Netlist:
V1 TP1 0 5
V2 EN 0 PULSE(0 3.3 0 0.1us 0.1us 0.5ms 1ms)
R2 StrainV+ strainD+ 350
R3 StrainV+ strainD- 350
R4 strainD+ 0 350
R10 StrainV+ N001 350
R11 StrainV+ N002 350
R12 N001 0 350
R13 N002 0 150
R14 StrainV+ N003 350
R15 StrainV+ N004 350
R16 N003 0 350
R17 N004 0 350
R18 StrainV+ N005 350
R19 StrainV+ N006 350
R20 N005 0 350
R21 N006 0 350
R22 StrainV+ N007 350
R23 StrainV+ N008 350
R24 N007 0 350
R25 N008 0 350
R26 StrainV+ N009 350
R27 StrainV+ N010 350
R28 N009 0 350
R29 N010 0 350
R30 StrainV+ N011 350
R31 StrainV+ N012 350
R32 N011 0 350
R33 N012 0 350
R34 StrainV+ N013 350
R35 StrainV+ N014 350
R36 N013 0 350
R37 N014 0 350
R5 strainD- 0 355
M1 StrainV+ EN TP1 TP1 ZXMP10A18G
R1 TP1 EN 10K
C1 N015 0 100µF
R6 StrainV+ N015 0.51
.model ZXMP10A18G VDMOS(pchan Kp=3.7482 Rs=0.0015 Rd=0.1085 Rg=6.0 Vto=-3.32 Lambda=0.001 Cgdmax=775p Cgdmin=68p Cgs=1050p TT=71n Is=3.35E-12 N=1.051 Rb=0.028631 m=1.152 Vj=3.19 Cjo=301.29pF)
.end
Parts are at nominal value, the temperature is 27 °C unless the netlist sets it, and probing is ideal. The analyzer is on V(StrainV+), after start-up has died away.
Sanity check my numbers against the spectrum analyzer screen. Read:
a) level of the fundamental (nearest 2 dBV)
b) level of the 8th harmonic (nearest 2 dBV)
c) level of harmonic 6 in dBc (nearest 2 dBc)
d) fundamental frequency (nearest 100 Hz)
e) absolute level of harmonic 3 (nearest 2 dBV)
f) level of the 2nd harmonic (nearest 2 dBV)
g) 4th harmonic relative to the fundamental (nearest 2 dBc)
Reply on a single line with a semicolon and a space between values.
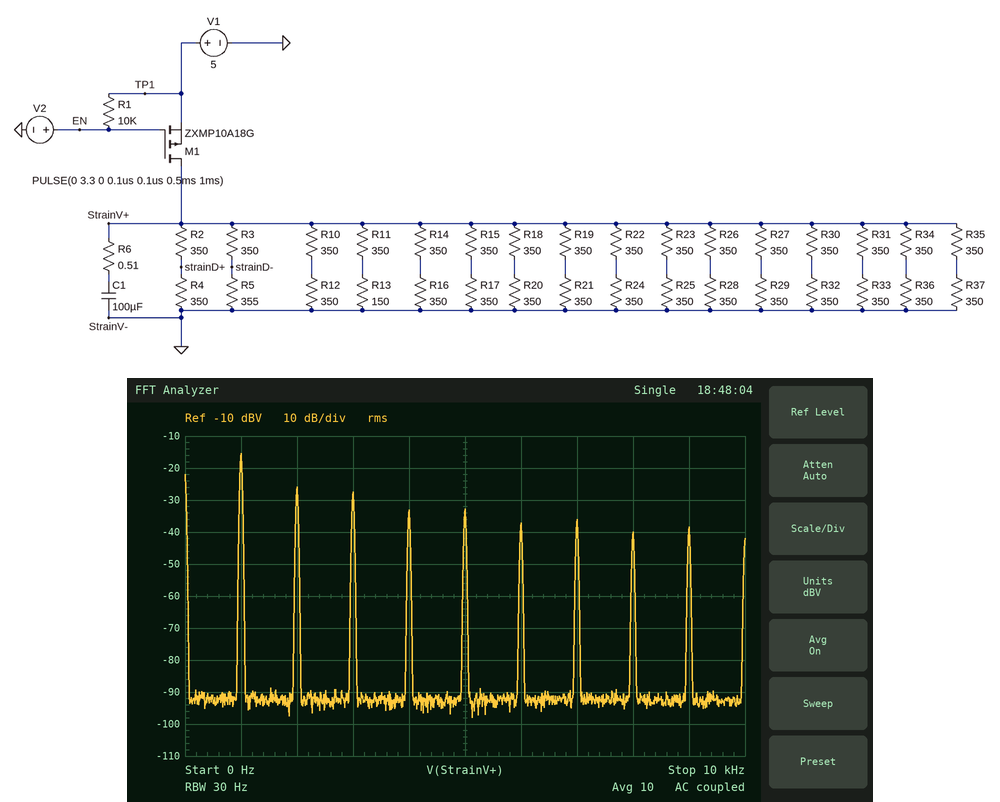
-16 dBV; -40 dBV; -22 dBc; 1.0 kHz; -28 dBV; -26 dBV; -18 dBc
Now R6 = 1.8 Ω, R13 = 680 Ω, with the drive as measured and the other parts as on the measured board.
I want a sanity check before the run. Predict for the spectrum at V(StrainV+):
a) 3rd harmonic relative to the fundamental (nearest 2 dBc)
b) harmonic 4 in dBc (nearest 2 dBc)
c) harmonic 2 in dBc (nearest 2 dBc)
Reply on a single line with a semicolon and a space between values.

-10 dBc; -20 dBc; -14 dBc
